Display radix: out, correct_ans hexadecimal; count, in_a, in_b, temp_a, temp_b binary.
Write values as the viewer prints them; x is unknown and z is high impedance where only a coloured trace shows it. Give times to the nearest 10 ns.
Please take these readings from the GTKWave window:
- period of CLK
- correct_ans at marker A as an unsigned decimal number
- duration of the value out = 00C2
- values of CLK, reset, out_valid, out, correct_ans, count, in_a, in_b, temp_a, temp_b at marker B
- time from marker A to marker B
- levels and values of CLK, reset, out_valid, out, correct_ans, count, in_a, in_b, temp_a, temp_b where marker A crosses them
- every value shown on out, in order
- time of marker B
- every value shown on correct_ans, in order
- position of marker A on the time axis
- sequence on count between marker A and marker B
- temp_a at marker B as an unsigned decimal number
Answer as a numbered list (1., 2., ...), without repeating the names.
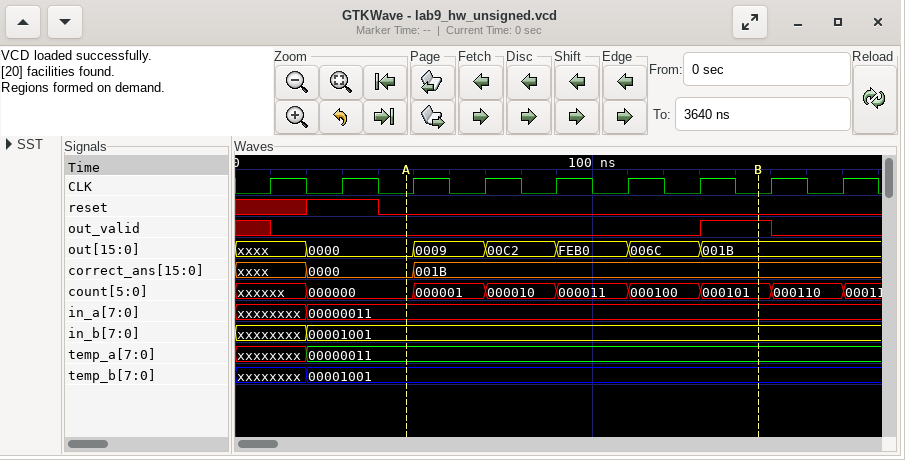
1. 20 ns
2. 0
3. 20 ns
4. CLK=0, reset=0, out_valid=1, out=001B, correct_ans=001B, count=000101, in_a=00000011, in_b=00001001, temp_a=00000011, temp_b=00001001
5. 100 ns
6. CLK=0, reset=0, out_valid=0, out=0000, correct_ans=0000, count=000000, in_a=00000011, in_b=00001001, temp_a=00000011, temp_b=00001001
7. xxxx, 0000, 0009, 00C2, FEB0, 006C, 001B
8. 150 ns
9. xxxx, 0000, 001B
10. 50 ns
11. 000000, 000001, 000010, 000011, 000100, 000101
12. 3
